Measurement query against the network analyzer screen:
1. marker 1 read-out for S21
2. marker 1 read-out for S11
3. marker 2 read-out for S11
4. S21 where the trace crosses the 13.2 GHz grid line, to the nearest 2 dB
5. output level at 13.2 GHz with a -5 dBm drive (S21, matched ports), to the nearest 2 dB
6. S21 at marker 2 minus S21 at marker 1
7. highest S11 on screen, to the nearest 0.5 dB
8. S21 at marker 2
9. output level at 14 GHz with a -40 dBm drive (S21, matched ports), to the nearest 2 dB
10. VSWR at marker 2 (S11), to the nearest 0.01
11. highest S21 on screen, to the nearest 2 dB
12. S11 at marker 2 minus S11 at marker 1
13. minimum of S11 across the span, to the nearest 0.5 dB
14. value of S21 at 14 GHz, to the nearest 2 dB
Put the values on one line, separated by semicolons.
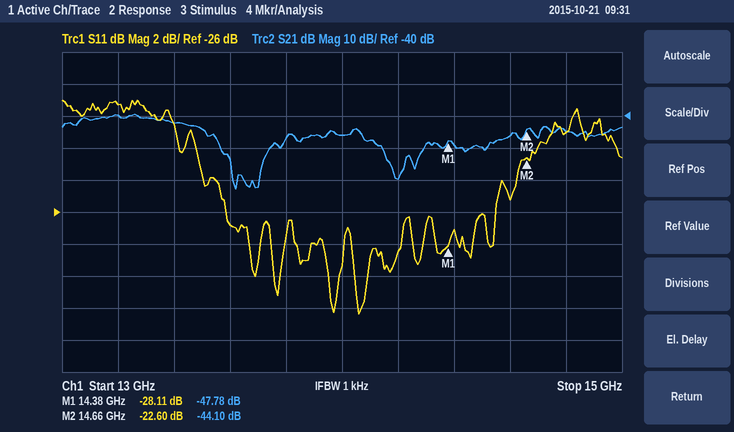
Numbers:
-47.78 dB; -28.11 dB; -22.60 dB; -40 dB; -44 dBm; 3.68 dB; -19.0 dB; -44.10 dB; -86 dBm; 1.16; -40 dB; 5.51 dB; -32.5 dB; -46 dB
